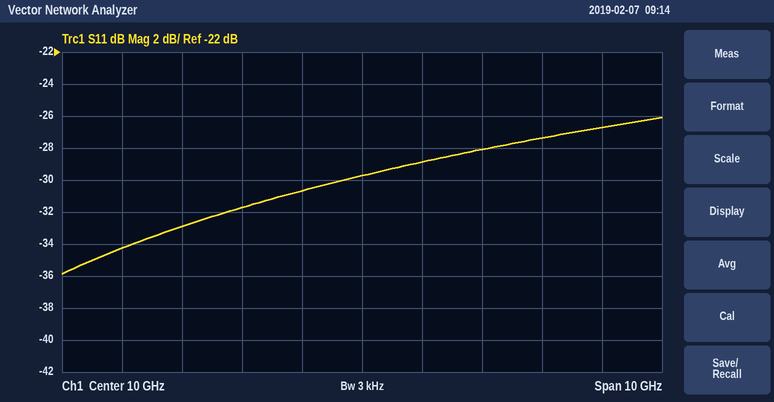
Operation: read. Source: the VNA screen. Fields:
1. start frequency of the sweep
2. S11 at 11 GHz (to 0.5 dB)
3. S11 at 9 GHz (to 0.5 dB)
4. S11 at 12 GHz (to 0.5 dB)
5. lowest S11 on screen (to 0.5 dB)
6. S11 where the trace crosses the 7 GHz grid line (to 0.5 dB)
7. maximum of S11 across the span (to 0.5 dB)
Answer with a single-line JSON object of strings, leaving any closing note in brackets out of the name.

{"start frequency of the sweep": "5 GHz", "S11 at 11 GHz": "-29.0 dB", "S11 at 9 GHz": "-30.5 dB", "S11 at 12 GHz": "-28.0 dB", "lowest S11 on screen": "-36.0 dB", "S11 where the trace crosses the 7 GHz grid line": "-33.0 dB", "maximum of S11 across the span": "-26.0 dB"}
